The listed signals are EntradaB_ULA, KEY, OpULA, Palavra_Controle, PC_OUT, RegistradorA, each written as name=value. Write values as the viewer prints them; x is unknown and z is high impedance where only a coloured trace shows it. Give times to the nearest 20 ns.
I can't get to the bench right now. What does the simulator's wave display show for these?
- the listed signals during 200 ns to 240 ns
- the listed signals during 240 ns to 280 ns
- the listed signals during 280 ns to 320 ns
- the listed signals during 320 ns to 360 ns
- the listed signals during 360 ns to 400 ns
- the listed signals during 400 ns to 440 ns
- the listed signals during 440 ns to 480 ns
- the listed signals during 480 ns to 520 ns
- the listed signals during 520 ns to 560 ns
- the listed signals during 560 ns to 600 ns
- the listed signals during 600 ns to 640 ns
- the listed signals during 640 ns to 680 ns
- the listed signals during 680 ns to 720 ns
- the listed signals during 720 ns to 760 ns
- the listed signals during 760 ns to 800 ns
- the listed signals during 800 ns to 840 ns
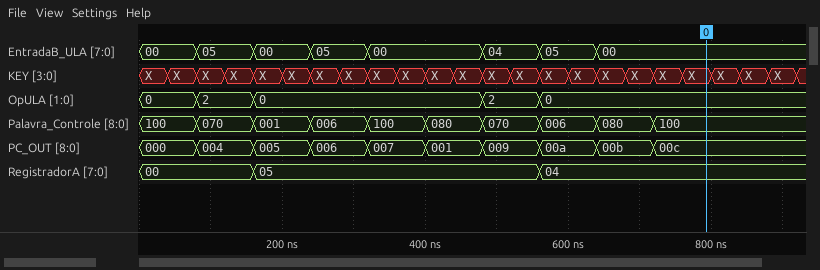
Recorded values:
EntradaB_ULA=00, KEY=X, OpULA=0, Palavra_Controle=001, PC_OUT=005, RegistradorA=05
EntradaB_ULA=05, KEY=X, OpULA=0, Palavra_Controle=006, PC_OUT=006, RegistradorA=05
EntradaB_ULA=05, KEY=X, OpULA=0, Palavra_Controle=006, PC_OUT=006, RegistradorA=05
EntradaB_ULA=00, KEY=X, OpULA=0, Palavra_Controle=100, PC_OUT=007, RegistradorA=05
EntradaB_ULA=00, KEY=X, OpULA=0, Palavra_Controle=100, PC_OUT=007, RegistradorA=05
EntradaB_ULA=00, KEY=X, OpULA=0, Palavra_Controle=080, PC_OUT=001, RegistradorA=05
EntradaB_ULA=00, KEY=X, OpULA=0, Palavra_Controle=080, PC_OUT=001, RegistradorA=05
EntradaB_ULA=04, KEY=X, OpULA=2, Palavra_Controle=070, PC_OUT=009, RegistradorA=05
EntradaB_ULA=04, KEY=X, OpULA=2, Palavra_Controle=070, PC_OUT=009, RegistradorA=05
EntradaB_ULA=05, KEY=X, OpULA=0, Palavra_Controle=006, PC_OUT=00a, RegistradorA=04
EntradaB_ULA=05, KEY=X, OpULA=0, Palavra_Controle=006, PC_OUT=00a, RegistradorA=04
EntradaB_ULA=00, KEY=X, OpULA=0, Palavra_Controle=080, PC_OUT=00b, RegistradorA=04
EntradaB_ULA=00, KEY=X, OpULA=0, Palavra_Controle=080, PC_OUT=00b, RegistradorA=04
EntradaB_ULA=00, KEY=X, OpULA=0, Palavra_Controle=100, PC_OUT=00c, RegistradorA=04
EntradaB_ULA=00, KEY=X, OpULA=0, Palavra_Controle=100, PC_OUT=00c, RegistradorA=04
EntradaB_ULA=00, KEY=X, OpULA=0, Palavra_Controle=100, PC_OUT=00c, RegistradorA=04
